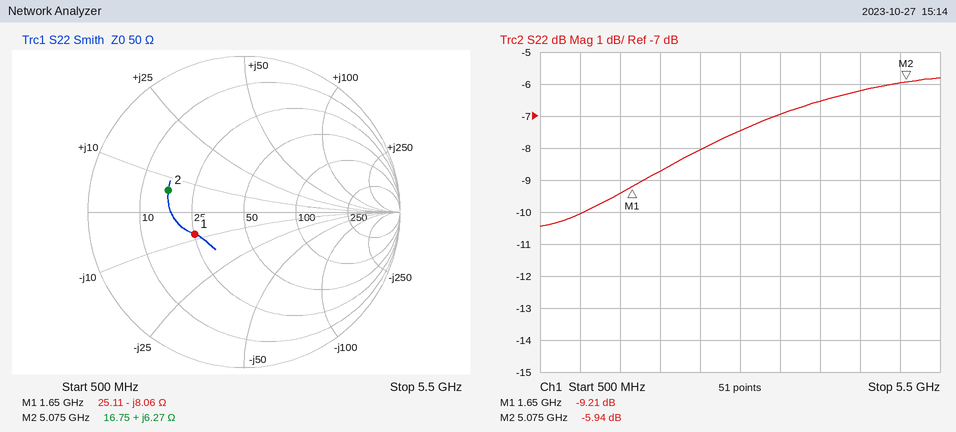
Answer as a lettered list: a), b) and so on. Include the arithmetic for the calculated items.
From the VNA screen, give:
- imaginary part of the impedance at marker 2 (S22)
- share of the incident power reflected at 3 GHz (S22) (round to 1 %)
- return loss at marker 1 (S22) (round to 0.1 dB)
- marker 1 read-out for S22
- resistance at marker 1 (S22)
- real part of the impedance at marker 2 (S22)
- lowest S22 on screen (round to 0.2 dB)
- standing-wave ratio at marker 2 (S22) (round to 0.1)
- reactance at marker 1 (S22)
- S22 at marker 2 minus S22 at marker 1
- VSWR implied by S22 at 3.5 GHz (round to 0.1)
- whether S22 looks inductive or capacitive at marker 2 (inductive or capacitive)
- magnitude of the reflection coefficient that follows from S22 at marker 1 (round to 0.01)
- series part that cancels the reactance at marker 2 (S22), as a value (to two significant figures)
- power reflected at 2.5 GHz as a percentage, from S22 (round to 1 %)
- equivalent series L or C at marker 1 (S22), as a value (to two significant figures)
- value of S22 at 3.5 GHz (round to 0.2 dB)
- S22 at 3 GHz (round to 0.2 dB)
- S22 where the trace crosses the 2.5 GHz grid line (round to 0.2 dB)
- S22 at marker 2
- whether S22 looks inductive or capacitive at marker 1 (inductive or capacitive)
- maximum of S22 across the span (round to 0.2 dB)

a) +6.27 Ω
b) 10^(-7.4/10) ≈ 18 %
c) 9.2 dB
d) -9.21 dB
e) 25.11 Ω
f) 16.75 Ω
g) -10.4 dB
h) 3.0
i) -8.06 Ω
j) -5.94 − (-9.21) = 3.27 dB
k) |Γ| = 10^(-7/20) = 0.4467; VSWR = (1 + 0.4467)/(1 − 0.4467) ≈ 2.6
l) inductive
m) 10^(-9.21/20) ≈ 0.35
n) C = 1/(2π × 5.075 GHz × 6.27 Ω) ≈ 5.0 pF
o) 10^(-8/10) ≈ 16 %
p) C = 1/(2π × 1.65 GHz × 8.06 Ω) ≈ 12 pF
q) -7.0 dB
r) -7.4 dB
s) -8.0 dB
t) -5.94 dB
u) capacitive
v) -5.8 dB
